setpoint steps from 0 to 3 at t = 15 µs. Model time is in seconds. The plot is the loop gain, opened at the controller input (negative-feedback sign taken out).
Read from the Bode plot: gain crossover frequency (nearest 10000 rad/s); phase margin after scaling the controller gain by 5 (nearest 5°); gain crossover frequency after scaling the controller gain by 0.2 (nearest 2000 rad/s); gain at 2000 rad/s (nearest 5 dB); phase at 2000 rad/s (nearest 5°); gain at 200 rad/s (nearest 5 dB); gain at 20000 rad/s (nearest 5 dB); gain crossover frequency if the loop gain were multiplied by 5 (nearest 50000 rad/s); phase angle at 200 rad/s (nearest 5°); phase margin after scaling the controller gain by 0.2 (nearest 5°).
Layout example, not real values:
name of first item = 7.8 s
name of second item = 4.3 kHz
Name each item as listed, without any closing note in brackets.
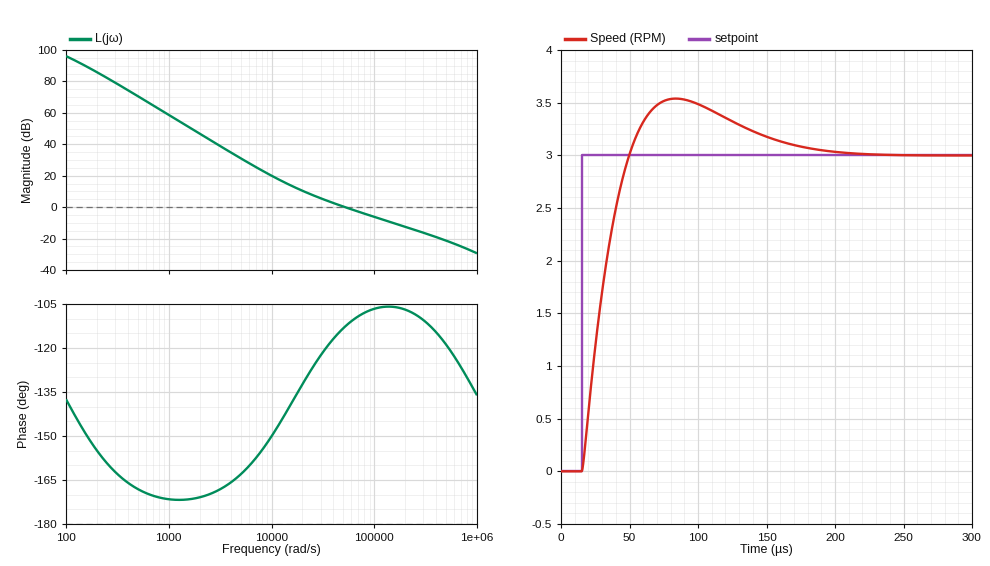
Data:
gain crossover frequency = 50000 rad/s
phase margin after scaling the controller gain by 5 = 70°
gain crossover frequency after scaling the controller gain by 0.2 = 16000 rad/s
gain at 2000 rad/s = 45 dB
phase at 2000 rad/s = -170°
gain at 200 rad/s = 85 dB
gain at 20000 rad/s = 10 dB
gain crossover frequency if the loop gain were multiplied by 5 = 250000 rad/s
phase angle at 200 rad/s = -155°
phase margin after scaling the controller gain by 0.2 = 40°
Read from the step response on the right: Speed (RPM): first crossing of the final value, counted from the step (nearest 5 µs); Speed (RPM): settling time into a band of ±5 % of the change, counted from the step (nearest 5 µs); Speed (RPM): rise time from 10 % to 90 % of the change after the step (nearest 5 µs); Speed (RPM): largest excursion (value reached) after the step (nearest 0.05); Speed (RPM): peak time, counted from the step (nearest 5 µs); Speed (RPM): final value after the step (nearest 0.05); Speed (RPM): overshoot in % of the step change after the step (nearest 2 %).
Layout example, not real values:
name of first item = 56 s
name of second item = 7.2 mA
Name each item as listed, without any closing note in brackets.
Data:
Speed (RPM): first crossing of the final value, counted from the step = 35 µs
Speed (RPM): settling time into a band of ±5 % of the change, counted from the step = 140 µs
Speed (RPM): rise time from 10 % to 90 % of the change after the step = 25 µs
Speed (RPM): largest excursion (value reached) after the step = 3.55
Speed (RPM): peak time, counted from the step = 70 µs
Speed (RPM): final value after the step = 3.00
Speed (RPM): overshoot in % of the step change after the step = 18 %
